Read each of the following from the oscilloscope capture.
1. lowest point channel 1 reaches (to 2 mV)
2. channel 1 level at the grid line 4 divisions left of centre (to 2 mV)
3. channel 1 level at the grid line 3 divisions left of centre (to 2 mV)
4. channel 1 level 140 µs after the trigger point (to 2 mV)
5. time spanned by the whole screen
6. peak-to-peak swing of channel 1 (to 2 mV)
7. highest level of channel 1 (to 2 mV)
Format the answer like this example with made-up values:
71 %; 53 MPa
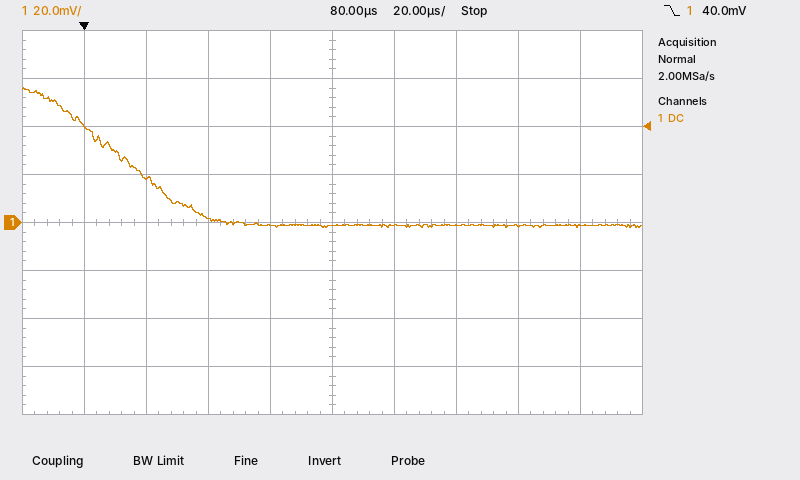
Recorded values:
-2 mV; 40 mV; 18 mV; -2 mV; 200 µs; 58 mV; 56 mV
